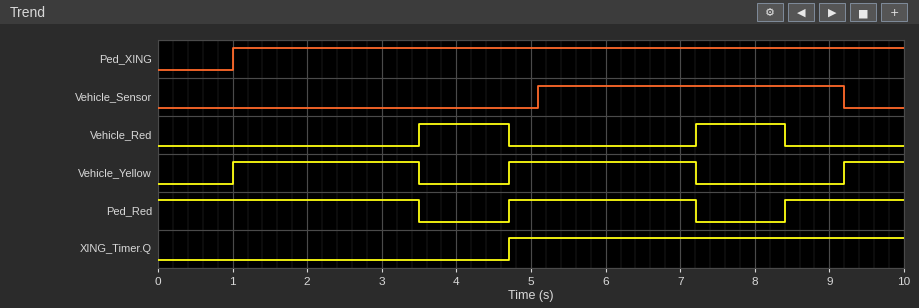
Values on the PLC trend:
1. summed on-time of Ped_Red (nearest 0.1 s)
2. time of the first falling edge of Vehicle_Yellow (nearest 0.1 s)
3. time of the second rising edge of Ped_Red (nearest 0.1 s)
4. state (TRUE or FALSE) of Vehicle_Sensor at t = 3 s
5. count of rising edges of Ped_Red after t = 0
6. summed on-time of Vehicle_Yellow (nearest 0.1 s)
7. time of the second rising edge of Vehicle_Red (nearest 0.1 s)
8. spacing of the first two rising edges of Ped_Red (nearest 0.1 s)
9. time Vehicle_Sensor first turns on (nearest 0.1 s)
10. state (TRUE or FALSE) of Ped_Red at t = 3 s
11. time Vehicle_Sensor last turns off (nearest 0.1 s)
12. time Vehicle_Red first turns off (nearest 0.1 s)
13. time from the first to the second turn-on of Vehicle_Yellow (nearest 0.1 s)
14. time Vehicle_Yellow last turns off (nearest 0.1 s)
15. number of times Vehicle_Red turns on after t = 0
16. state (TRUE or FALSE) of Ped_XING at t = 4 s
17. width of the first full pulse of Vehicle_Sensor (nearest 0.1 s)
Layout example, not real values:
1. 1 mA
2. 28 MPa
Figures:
1. 7.6 s
2. 3.5 s
3. 8.4 s
4. FALSE
5. 2
6. 5.8 s
7. 7.2 s
8. 3.7 s
9. 5.1 s
10. TRUE
11. 9.2 s
12. 4.7 s
13. 3.7 s
14. 7.2 s
15. 2
16. TRUE
17. 4.1 s
